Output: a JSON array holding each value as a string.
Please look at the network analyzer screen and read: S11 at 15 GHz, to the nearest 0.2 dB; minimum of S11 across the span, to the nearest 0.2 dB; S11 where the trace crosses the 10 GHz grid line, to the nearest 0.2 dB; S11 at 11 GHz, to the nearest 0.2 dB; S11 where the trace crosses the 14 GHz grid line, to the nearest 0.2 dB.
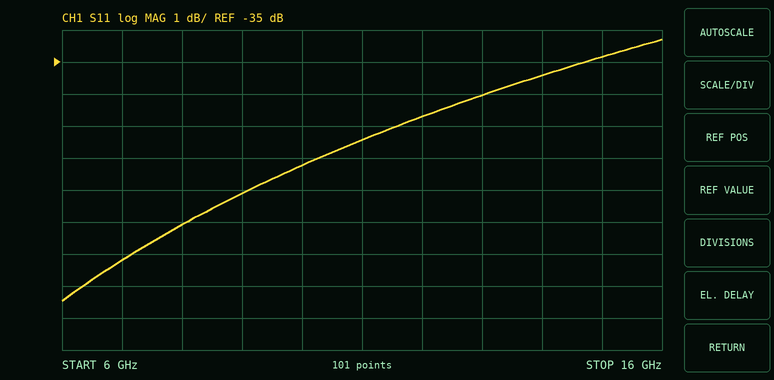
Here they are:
["-34.8 dB", "-42.4 dB", "-38.2 dB", "-37.4 dB", "-35.4 dB"]
